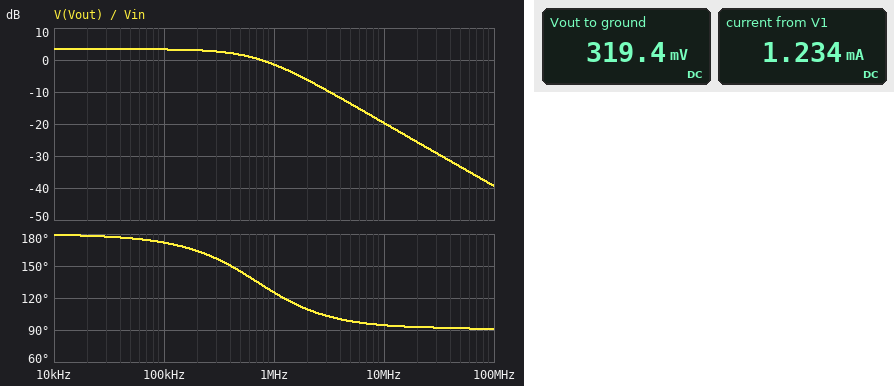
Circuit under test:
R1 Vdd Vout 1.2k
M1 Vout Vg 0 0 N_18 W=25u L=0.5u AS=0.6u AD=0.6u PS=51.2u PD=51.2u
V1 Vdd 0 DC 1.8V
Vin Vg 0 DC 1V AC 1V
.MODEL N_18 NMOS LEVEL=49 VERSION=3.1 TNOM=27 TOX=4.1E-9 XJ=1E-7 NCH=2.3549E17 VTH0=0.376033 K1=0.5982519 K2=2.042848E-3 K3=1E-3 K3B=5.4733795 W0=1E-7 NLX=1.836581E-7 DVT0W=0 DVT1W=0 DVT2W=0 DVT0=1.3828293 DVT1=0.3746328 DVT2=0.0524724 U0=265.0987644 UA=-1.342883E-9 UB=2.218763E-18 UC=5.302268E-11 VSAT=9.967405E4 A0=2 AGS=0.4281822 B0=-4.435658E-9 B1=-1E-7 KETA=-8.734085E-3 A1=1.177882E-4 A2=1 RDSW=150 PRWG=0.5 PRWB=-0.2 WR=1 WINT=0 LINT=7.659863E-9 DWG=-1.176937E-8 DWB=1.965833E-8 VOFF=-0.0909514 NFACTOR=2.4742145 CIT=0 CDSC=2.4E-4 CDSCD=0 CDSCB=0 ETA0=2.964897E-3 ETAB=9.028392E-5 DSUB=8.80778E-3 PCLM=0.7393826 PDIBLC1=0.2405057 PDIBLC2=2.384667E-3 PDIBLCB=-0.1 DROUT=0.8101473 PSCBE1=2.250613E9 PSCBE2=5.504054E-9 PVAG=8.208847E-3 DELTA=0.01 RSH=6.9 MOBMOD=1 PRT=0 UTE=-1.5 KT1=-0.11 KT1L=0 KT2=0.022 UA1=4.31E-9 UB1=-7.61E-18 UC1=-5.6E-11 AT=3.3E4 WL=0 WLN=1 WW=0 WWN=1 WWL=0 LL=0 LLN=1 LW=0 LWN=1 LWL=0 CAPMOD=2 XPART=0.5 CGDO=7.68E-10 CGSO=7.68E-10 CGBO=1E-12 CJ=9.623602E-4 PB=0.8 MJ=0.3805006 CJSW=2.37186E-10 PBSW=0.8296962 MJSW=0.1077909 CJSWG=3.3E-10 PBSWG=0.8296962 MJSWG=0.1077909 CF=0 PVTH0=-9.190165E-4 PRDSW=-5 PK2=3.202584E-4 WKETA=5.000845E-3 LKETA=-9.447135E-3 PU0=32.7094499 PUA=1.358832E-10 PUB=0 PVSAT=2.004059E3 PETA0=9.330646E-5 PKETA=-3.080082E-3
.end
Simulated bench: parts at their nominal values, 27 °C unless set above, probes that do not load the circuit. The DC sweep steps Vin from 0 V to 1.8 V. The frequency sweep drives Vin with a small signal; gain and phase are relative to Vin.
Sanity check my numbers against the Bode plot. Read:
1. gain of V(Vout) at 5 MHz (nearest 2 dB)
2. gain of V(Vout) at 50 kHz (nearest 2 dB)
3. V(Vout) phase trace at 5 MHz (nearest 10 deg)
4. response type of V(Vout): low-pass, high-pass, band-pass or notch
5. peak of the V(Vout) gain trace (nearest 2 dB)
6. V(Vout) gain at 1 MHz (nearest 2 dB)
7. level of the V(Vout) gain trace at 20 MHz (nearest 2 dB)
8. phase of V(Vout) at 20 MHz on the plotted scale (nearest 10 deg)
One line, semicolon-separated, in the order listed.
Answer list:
-14 dB; 4 dB; 100 deg; low-pass; 4 dB; -2 dB; -26 dB; 90 deg
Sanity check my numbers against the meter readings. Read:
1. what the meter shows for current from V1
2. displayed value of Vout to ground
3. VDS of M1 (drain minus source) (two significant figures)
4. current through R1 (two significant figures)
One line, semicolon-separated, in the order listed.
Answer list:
1.234 mA; 319.4 mV; 320 mV; 1.2 mA
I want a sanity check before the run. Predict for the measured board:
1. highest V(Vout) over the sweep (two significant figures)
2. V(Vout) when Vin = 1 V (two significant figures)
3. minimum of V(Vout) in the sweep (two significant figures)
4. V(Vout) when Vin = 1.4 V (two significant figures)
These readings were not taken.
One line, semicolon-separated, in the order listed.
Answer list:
1.8 V; 320 mV; 130 mV; 160 mV
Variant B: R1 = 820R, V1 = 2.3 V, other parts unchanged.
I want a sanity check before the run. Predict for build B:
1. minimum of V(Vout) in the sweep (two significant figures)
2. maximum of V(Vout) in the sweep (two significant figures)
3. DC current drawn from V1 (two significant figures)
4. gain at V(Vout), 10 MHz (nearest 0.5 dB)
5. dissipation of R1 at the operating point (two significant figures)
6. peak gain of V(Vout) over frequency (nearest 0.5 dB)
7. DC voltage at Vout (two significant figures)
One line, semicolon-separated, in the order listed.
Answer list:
240 mV; 2.3 V; 1.4 mA; -15.5 dB; 1.6 mW; 11.0 dB; 1.1 V
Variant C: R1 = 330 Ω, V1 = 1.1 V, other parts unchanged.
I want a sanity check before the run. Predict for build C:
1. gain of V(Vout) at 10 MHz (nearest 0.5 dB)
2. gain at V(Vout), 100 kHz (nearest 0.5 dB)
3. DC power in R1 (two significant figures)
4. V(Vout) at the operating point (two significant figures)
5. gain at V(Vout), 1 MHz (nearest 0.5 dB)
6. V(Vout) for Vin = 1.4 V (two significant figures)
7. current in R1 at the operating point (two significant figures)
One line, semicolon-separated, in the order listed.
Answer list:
-16.5 dB; 3.0 dB; 620 µW; 650 mV; 0 dB; 320 mV; 1.4 mA
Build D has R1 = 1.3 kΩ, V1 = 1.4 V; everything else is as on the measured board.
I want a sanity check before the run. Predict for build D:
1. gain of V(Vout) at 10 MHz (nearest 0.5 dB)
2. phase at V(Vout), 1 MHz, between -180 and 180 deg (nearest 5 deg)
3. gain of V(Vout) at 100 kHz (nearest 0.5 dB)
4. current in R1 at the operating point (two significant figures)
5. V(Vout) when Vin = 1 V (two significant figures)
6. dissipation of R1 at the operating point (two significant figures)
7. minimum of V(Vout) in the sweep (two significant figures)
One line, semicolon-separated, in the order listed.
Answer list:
-24.5 dB; 140 deg; -6.5 dB; 930 µA; 190 mV; 1.1 mW; 90 mV
